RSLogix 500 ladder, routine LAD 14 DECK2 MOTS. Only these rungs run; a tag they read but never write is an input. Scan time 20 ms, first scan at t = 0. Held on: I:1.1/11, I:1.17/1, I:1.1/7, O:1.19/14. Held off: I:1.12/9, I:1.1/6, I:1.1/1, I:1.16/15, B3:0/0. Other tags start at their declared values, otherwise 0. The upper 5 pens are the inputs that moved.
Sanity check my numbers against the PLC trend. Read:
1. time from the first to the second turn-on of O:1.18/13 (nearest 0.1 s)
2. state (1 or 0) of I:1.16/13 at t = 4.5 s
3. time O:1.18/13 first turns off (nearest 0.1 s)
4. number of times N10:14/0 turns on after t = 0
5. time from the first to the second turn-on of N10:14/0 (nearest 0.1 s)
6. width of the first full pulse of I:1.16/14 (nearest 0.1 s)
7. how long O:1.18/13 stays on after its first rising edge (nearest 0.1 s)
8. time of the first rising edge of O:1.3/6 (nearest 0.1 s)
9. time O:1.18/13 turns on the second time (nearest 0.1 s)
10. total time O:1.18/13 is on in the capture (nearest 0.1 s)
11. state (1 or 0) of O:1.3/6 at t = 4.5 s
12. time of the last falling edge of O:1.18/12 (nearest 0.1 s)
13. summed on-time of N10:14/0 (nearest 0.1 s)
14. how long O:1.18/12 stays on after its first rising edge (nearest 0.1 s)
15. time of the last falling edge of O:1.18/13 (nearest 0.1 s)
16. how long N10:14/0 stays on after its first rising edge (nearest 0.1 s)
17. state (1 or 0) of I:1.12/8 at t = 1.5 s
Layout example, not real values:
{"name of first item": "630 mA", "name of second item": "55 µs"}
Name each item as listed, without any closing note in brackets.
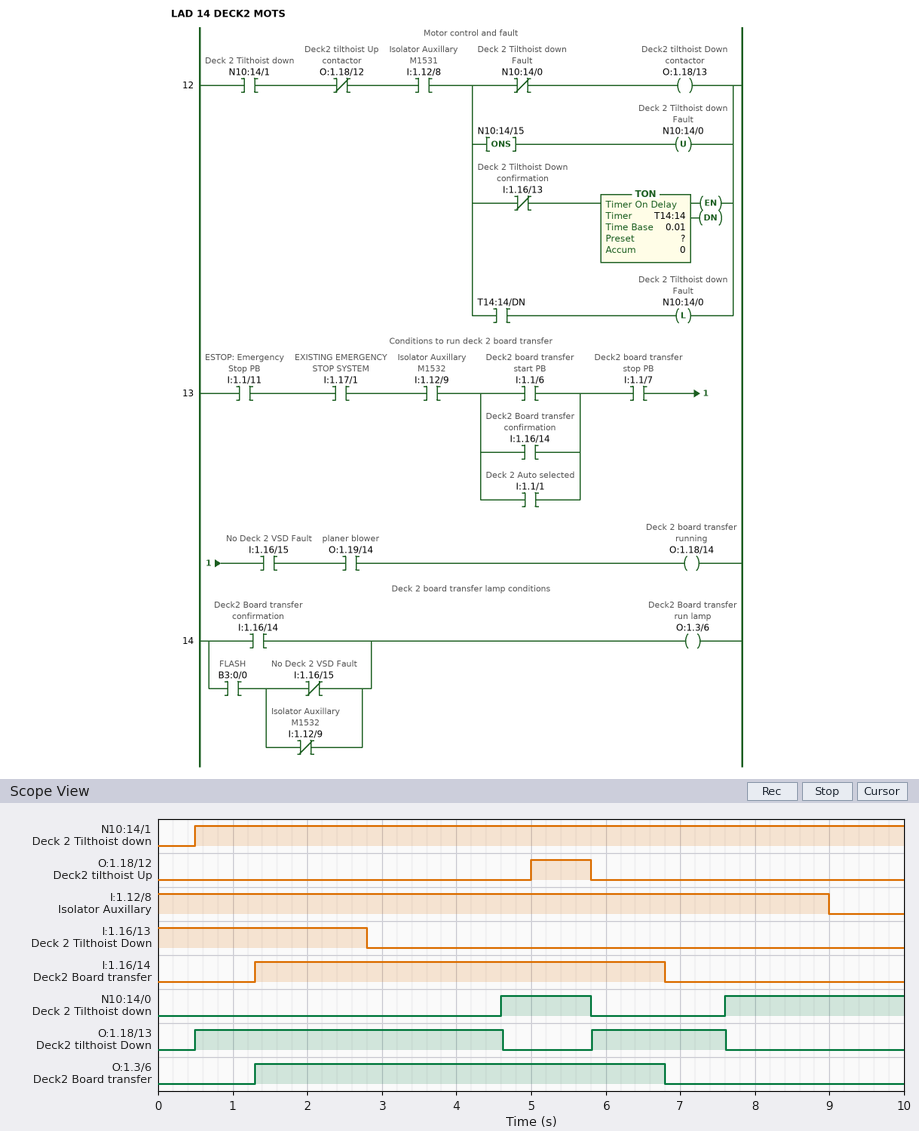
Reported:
{"time from the first to the second turn-on of O:1.18/13": "5.3 s", "state (1 or 0) of I:1.16/13 at t = 4.5 s": "0", "time O:1.18/13 first turns off": "4.6 s", "number of times N10:14/0 turns on after t = 0": "2", "time from the first to the second turn-on of N10:14/0": "3.0 s", "width of the first full pulse of I:1.16/14": "5.5 s", "how long O:1.18/13 stays on after its first rising edge": "4.1 s", "time of the first rising edge of O:1.3/6": "1.3 s", "time O:1.18/13 turns on the second time": "5.8 s", "total time O:1.18/13 is on in the capture": "5.9 s", "state (1 or 0) of O:1.3/6 at t = 4.5 s": "1", "time of the last falling edge of O:1.18/12": "5.8 s", "summed on-time of N10:14/0": "3.6 s", "how long O:1.18/12 stays on after its first rising edge": "0.8 s", "time of the last falling edge of O:1.18/13": "7.6 s", "how long N10:14/0 stays on after its first rising edge": "1.2 s", "state (1 or 0) of I:1.12/8 at t = 1.5 s": "1"}
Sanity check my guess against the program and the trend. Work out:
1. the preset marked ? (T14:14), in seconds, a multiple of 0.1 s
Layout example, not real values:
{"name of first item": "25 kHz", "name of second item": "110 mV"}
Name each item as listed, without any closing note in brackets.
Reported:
{"the preset marked ? (T14:14), in seconds, a multiple of 0.1 s": "1.8 s"}
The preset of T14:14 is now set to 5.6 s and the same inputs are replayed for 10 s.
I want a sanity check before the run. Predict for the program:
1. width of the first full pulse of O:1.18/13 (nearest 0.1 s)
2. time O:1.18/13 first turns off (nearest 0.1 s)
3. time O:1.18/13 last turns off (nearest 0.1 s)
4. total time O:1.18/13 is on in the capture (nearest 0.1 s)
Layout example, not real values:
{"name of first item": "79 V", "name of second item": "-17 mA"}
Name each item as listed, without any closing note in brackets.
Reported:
{"width of the first full pulse of O:1.18/13": "4.5 s", "time O:1.18/13 first turns off": "5.0 s", "time O:1.18/13 last turns off": "9.0 s", "total time O:1.18/13 is on in the capture": "7.7 s"}
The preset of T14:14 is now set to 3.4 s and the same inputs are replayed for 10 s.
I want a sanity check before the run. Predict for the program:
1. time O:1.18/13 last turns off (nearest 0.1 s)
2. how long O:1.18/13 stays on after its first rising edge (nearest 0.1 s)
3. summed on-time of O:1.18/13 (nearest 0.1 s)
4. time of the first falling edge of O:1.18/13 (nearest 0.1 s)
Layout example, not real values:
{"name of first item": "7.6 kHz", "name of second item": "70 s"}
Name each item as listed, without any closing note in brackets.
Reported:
{"time O:1.18/13 last turns off": "9.0 s", "how long O:1.18/13 stays on after its first rising edge": "4.5 s", "summed on-time of O:1.18/13": "7.7 s", "time of the first falling edge of O:1.18/13": "5.0 s"}
